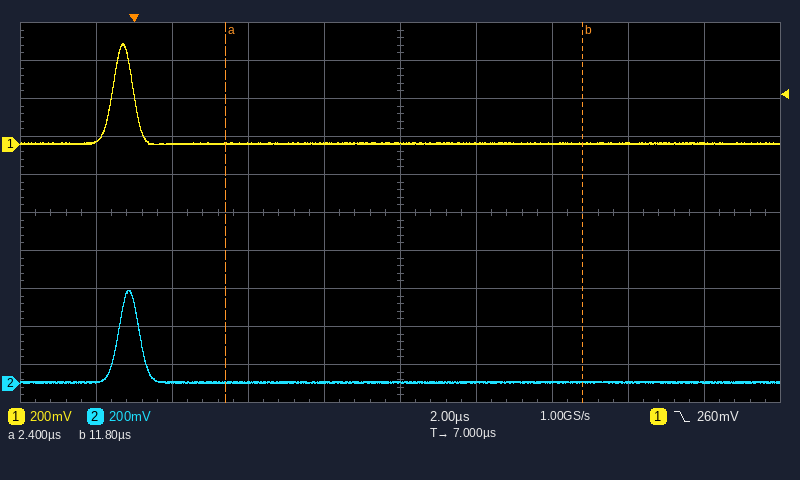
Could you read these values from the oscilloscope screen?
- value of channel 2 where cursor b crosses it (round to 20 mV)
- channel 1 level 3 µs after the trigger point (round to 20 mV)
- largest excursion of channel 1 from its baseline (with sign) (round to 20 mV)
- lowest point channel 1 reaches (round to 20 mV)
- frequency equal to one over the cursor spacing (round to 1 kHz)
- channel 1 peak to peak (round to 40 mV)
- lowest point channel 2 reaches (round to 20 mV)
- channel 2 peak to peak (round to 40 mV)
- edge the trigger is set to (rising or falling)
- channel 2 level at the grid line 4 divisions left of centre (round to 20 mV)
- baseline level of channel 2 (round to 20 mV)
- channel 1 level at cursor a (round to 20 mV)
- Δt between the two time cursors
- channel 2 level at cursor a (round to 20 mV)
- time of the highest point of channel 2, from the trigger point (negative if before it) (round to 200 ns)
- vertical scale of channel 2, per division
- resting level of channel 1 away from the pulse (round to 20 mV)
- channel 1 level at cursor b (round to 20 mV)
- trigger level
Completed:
0 mV
0 mV
+520 mV
0 mV
106 kHz
520 mV
0 mV
480 mV
falling
0 mV
0 mV
0 mV
9.4 µs
0 mV
-200 ns
200 mV
0 mV
0 mV
260 mV
